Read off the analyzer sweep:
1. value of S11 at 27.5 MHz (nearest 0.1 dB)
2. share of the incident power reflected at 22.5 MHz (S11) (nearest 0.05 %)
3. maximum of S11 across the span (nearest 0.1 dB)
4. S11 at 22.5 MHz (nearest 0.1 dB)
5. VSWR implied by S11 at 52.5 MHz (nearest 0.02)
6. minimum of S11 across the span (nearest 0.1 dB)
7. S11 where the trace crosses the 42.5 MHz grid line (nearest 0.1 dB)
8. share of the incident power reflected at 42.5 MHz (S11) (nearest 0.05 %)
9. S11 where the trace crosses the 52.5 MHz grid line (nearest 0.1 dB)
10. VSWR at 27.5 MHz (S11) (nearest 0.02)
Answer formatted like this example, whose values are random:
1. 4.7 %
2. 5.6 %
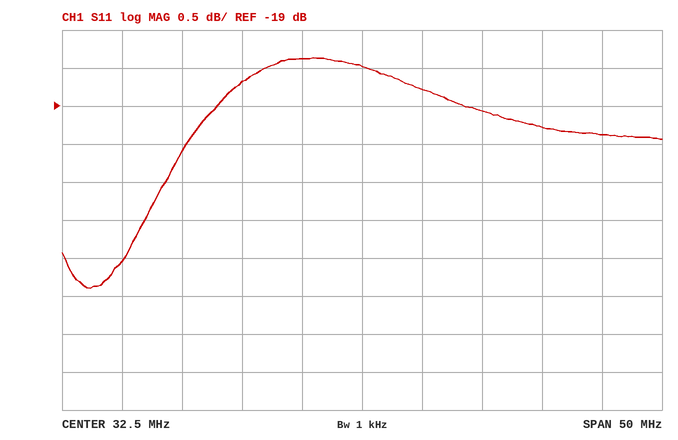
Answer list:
1. -18.4 dB
2. 1.35 %
3. -18.4 dB
4. -18.7 dB
5. 1.24
6. -21.4 dB
7. -19.1 dB
8. 1.25 %
9. -19.4 dB
10. 1.28
